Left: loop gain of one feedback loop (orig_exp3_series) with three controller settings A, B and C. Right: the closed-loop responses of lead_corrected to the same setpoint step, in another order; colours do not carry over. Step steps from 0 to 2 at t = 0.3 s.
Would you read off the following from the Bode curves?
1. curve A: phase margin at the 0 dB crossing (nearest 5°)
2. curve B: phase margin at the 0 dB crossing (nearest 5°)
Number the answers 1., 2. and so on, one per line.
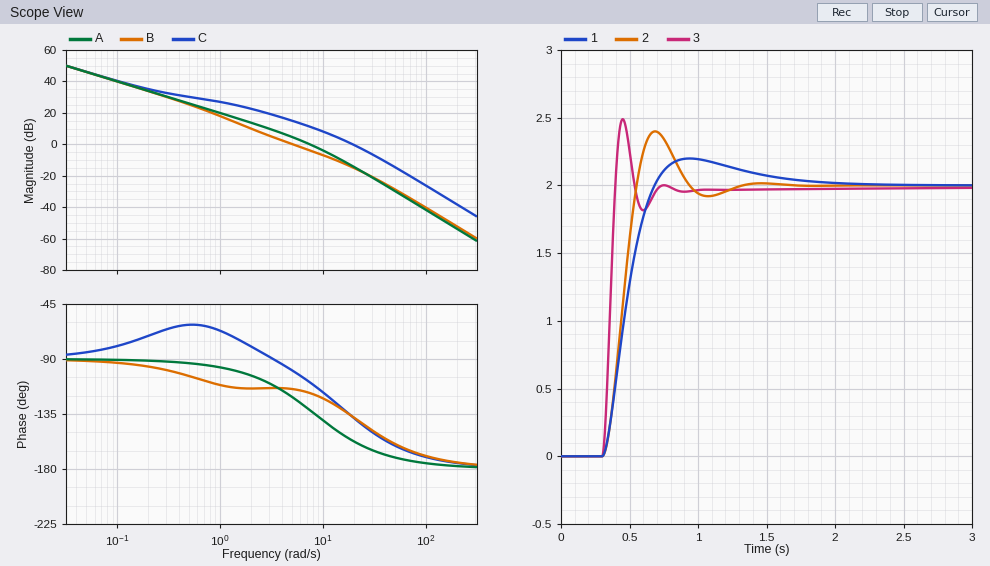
1. 50°
2. 65°
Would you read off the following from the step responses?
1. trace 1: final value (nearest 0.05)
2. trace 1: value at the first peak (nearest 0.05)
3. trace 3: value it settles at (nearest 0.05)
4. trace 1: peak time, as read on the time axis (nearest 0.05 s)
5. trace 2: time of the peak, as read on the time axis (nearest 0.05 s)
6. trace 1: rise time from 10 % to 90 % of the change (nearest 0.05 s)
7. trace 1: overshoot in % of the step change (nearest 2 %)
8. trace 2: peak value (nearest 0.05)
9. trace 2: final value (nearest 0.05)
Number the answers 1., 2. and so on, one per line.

1. 2.00
2. 2.20
3. 2.00
4. 0.95 s
5. 0.70 s
6. 0.25 s
7. 10 %
8. 2.40
9. 2.00
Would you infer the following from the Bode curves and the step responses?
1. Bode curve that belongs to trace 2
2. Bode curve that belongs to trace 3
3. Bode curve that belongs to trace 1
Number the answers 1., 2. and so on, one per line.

1. A
2. C
3. B
